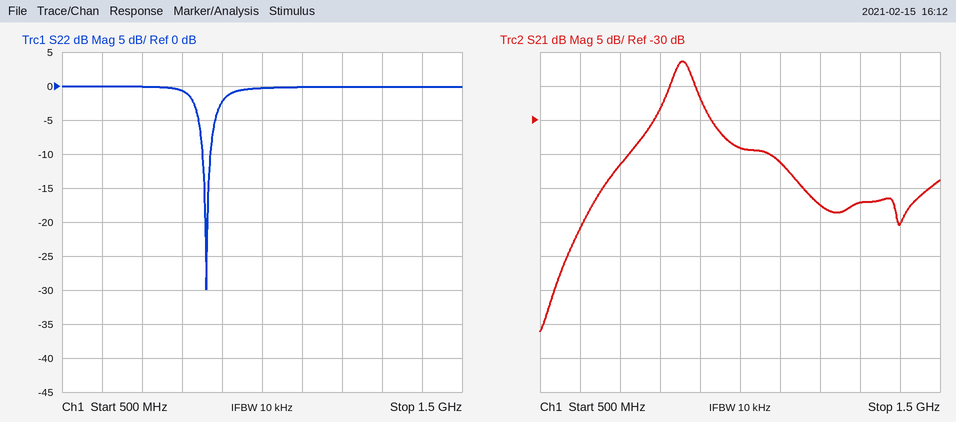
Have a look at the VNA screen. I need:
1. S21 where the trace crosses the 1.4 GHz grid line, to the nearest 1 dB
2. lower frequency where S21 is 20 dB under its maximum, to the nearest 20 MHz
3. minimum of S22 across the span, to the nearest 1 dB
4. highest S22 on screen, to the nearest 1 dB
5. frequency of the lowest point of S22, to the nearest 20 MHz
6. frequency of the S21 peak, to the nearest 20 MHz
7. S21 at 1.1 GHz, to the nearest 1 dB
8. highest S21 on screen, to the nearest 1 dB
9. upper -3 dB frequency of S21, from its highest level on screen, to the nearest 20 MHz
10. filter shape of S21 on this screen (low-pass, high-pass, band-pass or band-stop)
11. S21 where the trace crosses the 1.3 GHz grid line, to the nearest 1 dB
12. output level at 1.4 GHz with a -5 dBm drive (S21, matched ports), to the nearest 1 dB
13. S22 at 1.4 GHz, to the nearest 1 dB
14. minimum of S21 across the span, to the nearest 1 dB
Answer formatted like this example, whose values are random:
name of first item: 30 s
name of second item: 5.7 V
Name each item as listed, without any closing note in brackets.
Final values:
S21 where the trace crosses the 1.4 GHz grid line, to the nearest 1 dB: -45 dB
lower frequency where S21 is 20 dB under its maximum, to the nearest 20 MHz: 640 MHz
minimum of S22 across the span, to the nearest 1 dB: -30 dB
highest S22 on screen, to the nearest 1 dB: 0 dB
frequency of the lowest point of S22, to the nearest 20 MHz: 860 MHz
frequency of the S21 peak, to the nearest 20 MHz: 860 MHz
S21 at 1.1 GHz, to the nearest 1 dB: -36 dB
highest S21 on screen, to the nearest 1 dB: -21 dB
upper -3 dB frequency of S21, from its highest level on screen, to the nearest 20 MHz: 880 MHz
filter shape of S21 on this screen: band-pass
S21 where the trace crosses the 1.3 GHz grid line, to the nearest 1 dB: -42 dB
output level at 1.4 GHz with a -5 dBm drive (S21, matched ports), to the nearest 1 dB: -50 dBm
S22 at 1.4 GHz, to the nearest 1 dB: 0 dB
minimum of S21 across the span, to the nearest 1 dB: -61 dB
